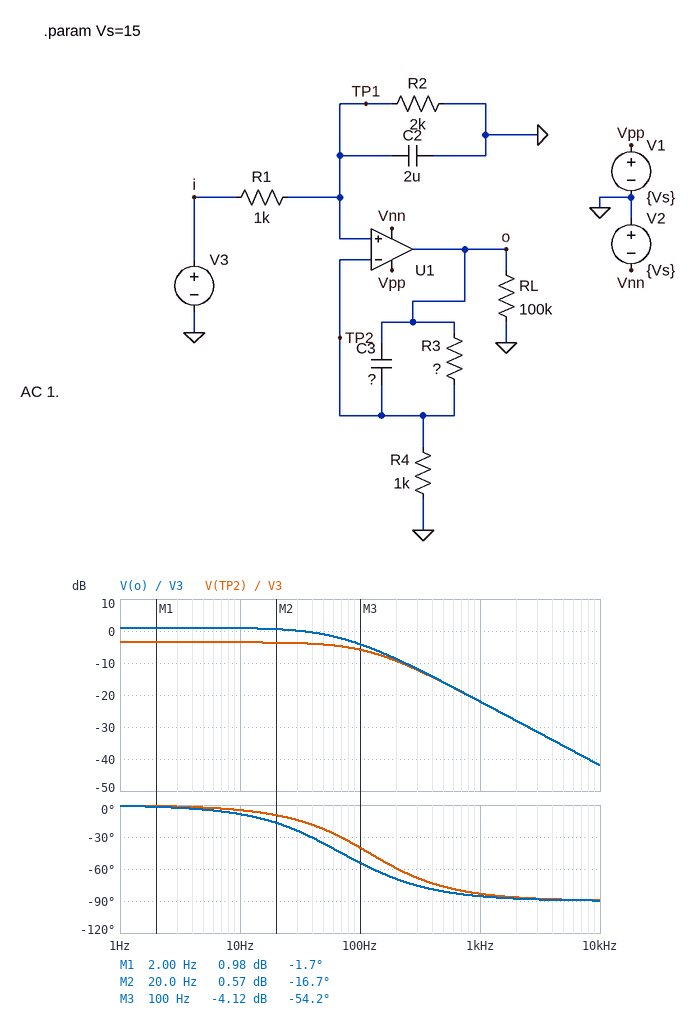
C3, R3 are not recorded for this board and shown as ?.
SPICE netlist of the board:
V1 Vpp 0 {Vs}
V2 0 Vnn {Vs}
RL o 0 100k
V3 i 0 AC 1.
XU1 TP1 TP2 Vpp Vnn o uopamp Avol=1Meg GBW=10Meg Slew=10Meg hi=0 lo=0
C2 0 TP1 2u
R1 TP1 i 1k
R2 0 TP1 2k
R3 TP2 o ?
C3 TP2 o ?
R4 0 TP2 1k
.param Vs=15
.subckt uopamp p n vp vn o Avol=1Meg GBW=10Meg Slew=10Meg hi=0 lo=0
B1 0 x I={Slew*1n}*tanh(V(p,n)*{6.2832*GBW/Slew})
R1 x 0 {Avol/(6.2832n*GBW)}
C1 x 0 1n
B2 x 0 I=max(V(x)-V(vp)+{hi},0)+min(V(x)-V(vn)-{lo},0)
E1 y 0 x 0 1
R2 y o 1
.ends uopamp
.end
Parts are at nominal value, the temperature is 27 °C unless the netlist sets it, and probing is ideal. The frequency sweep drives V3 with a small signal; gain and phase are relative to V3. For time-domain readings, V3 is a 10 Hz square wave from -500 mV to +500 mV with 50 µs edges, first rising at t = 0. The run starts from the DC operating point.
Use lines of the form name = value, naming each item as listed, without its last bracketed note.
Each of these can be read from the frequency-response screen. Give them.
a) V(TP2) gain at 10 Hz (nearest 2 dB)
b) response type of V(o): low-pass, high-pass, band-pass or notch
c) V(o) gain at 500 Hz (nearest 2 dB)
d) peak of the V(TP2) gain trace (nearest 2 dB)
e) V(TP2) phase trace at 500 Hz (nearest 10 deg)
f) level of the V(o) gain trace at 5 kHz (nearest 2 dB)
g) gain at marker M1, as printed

V(TP2) gain at 10 Hz = -4 dB
response type of V(o): low-pass, high-pass, band-pass or notch = low-pass
V(o) gain at 500 Hz = -16 dB
peak of the V(TP2) gain trace = -4 dB
V(TP2) phase trace at 500 Hz = -80 deg
level of the V(o) gain trace at 5 kHz = -36 dB
gain at marker M1, as printed = 0.98 dB
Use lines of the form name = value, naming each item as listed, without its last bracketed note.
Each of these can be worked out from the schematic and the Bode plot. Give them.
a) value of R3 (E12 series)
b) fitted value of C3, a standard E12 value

value of R3 = 680 Ω
fitted value of C3, a standard E12 value = 3.9 µF
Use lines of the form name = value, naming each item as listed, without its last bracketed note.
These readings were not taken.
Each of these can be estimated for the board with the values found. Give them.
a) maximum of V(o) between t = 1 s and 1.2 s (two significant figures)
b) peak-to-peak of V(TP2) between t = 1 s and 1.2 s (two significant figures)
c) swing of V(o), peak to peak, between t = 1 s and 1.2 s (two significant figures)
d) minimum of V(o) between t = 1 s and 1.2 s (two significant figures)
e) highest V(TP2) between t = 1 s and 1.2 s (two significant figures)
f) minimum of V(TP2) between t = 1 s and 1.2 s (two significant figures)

maximum of V(o) between t = 1 s and 1.2 s = 560 mV
peak-to-peak of V(TP2) between t = 1 s and 1.2 s = 670 mV
swing of V(o), peak to peak, between t = 1 s and 1.2 s = 1.1 V
minimum of V(o) between t = 1 s and 1.2 s = -560 mV
highest V(TP2) between t = 1 s and 1.2 s = 330 mV
minimum of V(TP2) between t = 1 s and 1.2 s = -330 mV
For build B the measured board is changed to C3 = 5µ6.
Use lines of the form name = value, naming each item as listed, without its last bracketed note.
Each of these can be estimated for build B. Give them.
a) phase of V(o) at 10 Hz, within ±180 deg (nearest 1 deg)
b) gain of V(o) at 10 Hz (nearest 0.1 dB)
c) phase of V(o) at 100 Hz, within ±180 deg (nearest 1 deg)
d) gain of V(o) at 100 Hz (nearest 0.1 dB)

phase of V(o) at 10 Hz, within ±180 deg = -10 deg
gain of V(o) at 10 Hz = 0.8 dB
phase of V(o) at 100 Hz, within ±180 deg = -52 deg
gain of V(o) at 100 Hz = -4.8 dB
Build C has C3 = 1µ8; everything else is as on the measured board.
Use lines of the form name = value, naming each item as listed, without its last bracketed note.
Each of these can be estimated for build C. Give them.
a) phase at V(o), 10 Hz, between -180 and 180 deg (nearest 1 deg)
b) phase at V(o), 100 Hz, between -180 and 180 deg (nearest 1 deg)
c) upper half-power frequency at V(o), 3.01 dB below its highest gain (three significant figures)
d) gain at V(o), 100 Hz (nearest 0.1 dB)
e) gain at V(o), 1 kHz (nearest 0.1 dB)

phase at V(o), 10 Hz, between -180 and 180 deg = -7 deg
phase at V(o), 100 Hz, between -180 and 180 deg = -53 deg
upper half-power frequency at V(o), 3.01 dB below its highest gain = 90.7 Hz
gain at V(o), 100 Hz = -2.5 dB
gain at V(o), 1 kHz = -21.9 dB
